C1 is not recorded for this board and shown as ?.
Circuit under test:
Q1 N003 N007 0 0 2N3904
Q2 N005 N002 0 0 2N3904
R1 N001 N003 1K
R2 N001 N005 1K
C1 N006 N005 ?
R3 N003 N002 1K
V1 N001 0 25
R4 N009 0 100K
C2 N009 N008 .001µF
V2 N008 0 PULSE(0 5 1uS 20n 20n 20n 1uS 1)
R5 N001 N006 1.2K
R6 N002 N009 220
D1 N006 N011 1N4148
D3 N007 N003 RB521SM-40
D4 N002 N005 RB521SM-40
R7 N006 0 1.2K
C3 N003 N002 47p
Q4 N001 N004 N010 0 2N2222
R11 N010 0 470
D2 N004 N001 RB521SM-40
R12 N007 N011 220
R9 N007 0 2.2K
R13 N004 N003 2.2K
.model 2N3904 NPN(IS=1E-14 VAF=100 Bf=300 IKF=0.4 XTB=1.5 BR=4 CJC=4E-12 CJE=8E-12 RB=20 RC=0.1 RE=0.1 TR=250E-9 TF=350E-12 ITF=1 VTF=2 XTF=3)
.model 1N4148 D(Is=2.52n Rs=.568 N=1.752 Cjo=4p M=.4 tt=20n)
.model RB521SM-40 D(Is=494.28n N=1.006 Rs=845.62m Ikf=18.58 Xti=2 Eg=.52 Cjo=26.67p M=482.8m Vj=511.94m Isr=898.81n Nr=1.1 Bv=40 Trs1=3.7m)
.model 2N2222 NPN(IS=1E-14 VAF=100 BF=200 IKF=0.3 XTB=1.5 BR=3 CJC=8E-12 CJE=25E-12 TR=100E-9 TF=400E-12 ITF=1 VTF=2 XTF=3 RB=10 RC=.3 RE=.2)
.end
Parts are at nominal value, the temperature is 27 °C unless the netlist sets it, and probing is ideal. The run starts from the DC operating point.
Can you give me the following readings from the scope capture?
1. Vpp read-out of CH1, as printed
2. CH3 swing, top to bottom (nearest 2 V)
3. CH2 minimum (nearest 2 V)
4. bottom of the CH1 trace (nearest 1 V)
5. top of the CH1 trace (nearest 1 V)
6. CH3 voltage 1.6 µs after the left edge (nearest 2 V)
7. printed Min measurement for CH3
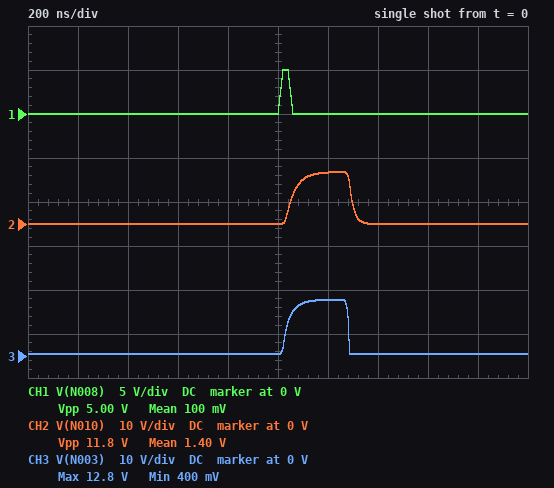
5.00 V
12 V
0 V
0 V
5 V
0 V
400 mV
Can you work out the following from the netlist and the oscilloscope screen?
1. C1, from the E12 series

390 pF
